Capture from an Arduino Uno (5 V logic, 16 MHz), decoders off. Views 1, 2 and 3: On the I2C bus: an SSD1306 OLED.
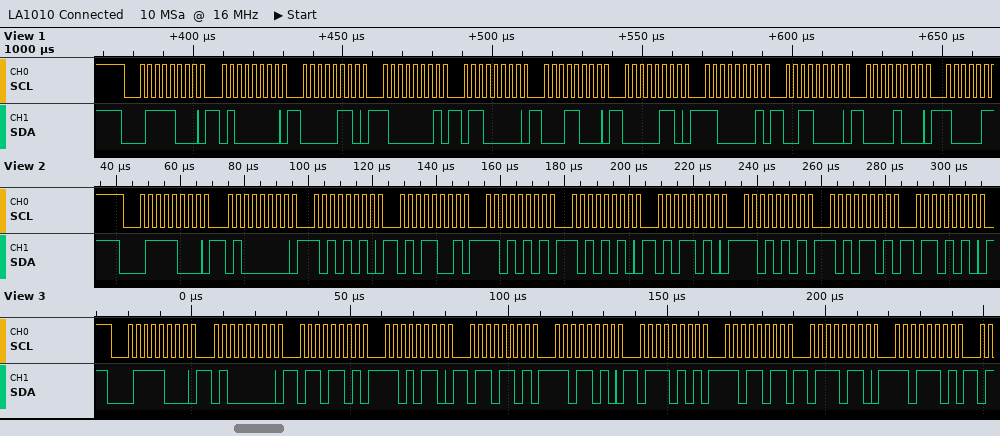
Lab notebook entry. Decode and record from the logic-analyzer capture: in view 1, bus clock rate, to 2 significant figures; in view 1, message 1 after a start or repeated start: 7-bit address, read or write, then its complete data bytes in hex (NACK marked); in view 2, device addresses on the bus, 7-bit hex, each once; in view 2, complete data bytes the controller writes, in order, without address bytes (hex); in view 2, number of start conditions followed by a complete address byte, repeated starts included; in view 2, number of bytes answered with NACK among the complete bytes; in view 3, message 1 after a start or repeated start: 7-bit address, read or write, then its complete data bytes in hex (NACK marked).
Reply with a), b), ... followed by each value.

a) 400 kHz
b) 0x3C write: 40 06 81 60 18 06 C1 30 08
c) 0x3C
d) 40 AA 59 D5 AA 5A D5 AD 6A
e) 1
f) 0
g) 0x3C write: 40 6D D6 6D DA 75 DB 76 DD
